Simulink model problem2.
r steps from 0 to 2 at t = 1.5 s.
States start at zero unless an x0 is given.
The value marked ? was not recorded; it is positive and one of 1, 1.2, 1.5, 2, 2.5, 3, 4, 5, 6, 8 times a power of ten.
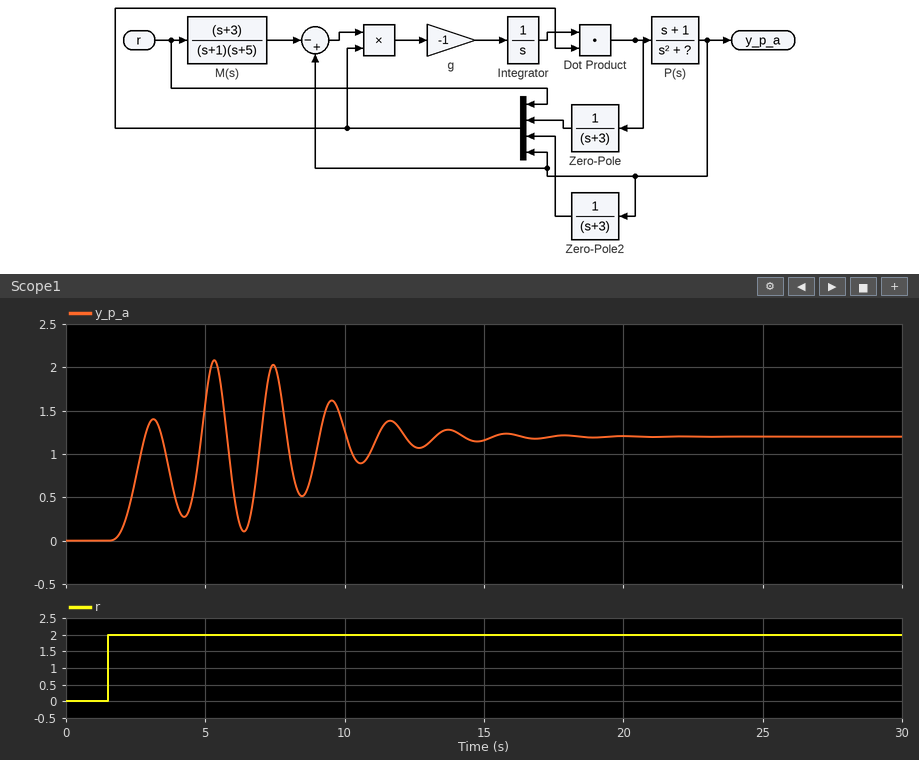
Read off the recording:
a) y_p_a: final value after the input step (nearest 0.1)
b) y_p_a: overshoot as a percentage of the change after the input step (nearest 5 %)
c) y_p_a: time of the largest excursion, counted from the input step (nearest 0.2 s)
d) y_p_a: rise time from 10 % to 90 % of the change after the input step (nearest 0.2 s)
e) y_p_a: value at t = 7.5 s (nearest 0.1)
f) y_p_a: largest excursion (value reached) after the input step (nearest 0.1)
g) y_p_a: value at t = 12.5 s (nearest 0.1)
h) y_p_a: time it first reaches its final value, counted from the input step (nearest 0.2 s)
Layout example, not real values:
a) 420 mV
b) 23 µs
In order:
a) 1.2
b) 75 %
c) 3.8 s
d) 0.8 s
e) 2.0
f) 2.1
g) 1.1
h) 1.4 s
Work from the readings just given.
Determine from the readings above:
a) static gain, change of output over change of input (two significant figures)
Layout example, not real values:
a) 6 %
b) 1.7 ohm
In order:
a) 0.60
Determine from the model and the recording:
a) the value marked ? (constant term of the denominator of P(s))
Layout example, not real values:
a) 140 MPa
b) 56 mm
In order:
a) 2
